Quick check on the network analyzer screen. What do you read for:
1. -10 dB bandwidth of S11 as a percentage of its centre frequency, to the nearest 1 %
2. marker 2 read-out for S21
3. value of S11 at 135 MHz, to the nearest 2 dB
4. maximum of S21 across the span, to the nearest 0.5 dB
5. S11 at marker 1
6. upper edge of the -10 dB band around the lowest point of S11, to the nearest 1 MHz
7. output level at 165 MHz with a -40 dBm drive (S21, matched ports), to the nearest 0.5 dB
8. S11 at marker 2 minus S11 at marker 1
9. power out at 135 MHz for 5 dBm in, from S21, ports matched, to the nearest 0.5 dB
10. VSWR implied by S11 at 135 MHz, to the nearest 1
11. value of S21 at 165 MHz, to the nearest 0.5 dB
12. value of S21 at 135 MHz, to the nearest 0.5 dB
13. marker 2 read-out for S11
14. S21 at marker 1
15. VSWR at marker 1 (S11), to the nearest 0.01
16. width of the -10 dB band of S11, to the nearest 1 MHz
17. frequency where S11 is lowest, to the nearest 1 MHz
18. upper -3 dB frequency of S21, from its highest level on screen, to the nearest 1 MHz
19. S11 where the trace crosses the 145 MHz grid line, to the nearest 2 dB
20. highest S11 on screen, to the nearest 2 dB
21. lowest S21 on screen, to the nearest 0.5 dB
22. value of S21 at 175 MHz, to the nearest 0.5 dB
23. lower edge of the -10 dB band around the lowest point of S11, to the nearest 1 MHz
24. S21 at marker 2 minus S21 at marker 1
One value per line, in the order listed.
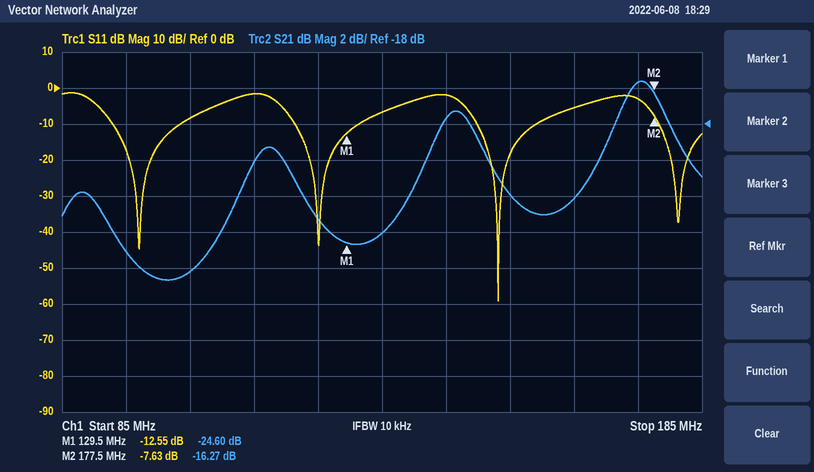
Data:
6 %
-16.27 dB
-6 dB
-15.5 dB
-12.55 dB
159 MHz
-62.0 dBm
4.92 dB
-19.0 dBm
3
-22.0 dB
-24.0 dB
-7.63 dB
-24.60 dB
1.62
9 MHz
153 MHz
181 MHz
-2 dB
-2 dB
-26.5 dB
-15.5 dB
150 MHz
8.33 dB
